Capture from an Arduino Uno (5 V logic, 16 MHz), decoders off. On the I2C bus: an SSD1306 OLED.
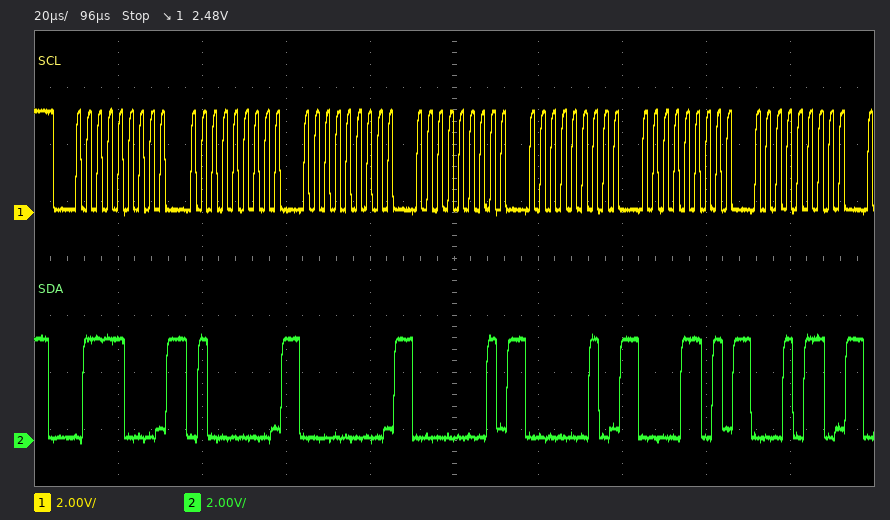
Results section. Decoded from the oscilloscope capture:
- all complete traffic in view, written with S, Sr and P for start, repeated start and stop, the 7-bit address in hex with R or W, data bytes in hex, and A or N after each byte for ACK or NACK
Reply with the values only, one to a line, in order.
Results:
S 3CW A 40 A 00 A 01 A 02 A 0D A 16 A
